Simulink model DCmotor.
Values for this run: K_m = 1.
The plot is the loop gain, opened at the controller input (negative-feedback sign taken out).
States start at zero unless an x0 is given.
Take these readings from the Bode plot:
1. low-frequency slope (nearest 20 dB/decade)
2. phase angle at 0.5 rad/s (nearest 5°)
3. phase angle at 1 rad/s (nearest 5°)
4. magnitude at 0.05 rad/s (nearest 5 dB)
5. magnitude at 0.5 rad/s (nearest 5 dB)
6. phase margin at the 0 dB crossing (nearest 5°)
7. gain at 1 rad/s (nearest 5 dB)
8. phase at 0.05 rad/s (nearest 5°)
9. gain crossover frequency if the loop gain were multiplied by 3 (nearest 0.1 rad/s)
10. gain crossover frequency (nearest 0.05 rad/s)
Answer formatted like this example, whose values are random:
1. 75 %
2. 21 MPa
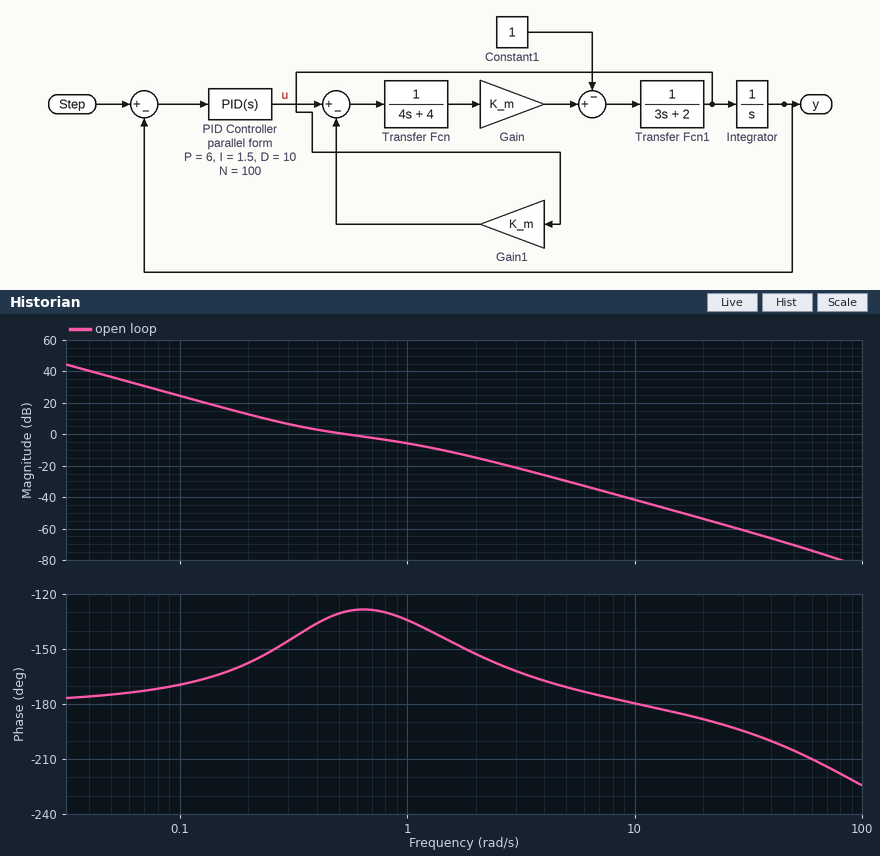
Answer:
1. -40 dB/decade
2. -130°
3. -135°
4. 35 dB
5. 0 dB
6. 50°
7. -5 dB
8. -175°
9. 1.4 rad/s
10. 0.55 rad/s
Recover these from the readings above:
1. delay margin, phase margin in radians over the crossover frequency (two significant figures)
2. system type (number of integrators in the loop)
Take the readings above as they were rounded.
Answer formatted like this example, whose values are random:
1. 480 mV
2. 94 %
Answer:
1. 1.6 s
2. 2
